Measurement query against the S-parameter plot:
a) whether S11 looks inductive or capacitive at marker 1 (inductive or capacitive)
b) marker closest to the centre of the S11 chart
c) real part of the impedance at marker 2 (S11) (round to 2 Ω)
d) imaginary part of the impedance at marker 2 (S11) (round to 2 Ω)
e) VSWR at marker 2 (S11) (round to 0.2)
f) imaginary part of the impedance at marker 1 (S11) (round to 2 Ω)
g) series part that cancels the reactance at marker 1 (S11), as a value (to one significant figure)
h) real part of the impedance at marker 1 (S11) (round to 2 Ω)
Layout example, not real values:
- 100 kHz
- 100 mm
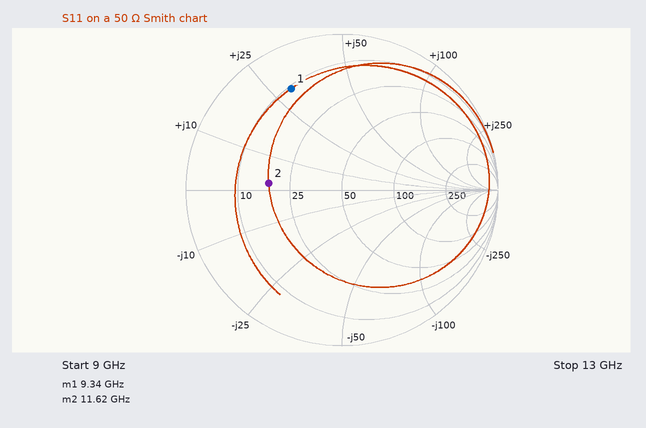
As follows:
- inductive
- marker 2
- 18 Ω
- +2 Ω
- 2.8
- +30 Ω
- 600 fF
- 10 Ω
